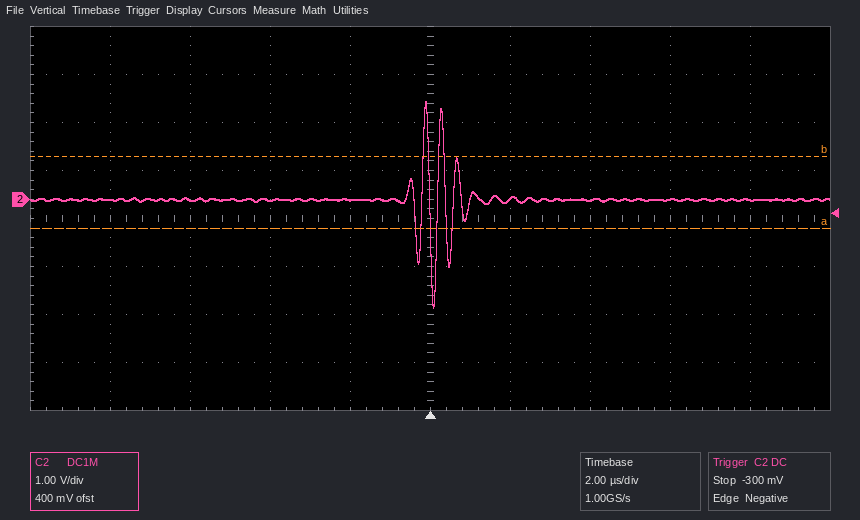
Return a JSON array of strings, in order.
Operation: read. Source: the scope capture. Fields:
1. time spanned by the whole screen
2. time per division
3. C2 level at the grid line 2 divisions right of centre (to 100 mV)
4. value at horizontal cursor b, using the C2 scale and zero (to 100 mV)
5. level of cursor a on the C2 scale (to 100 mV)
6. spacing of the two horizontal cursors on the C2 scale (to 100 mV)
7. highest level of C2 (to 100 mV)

["20 µs", "2 µs", "0.0 V", "900 mV", "-600 mV", "1.5 V", "2.0 V"]
